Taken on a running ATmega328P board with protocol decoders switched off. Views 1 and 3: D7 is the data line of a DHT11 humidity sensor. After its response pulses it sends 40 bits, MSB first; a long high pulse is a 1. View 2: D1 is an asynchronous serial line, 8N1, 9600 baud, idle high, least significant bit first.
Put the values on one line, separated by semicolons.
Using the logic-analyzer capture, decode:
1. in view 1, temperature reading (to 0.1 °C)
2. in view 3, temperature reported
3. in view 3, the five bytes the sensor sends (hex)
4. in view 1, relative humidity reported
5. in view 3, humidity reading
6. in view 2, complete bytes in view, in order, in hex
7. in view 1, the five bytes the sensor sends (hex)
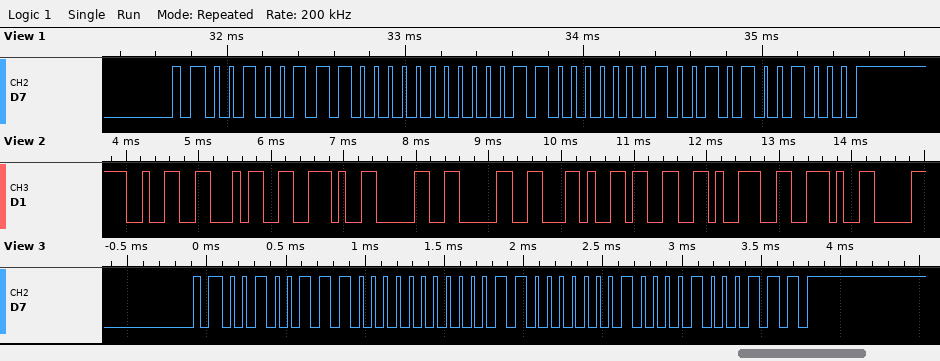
24.9 °C; 24.8 °C; 27 00 18 08 47; 39 %; 39 %; 0x32 0x34 0x2E 0x30 0x30 0x2C 0x33 0x39 0x2E; 27 00 18 09 48
